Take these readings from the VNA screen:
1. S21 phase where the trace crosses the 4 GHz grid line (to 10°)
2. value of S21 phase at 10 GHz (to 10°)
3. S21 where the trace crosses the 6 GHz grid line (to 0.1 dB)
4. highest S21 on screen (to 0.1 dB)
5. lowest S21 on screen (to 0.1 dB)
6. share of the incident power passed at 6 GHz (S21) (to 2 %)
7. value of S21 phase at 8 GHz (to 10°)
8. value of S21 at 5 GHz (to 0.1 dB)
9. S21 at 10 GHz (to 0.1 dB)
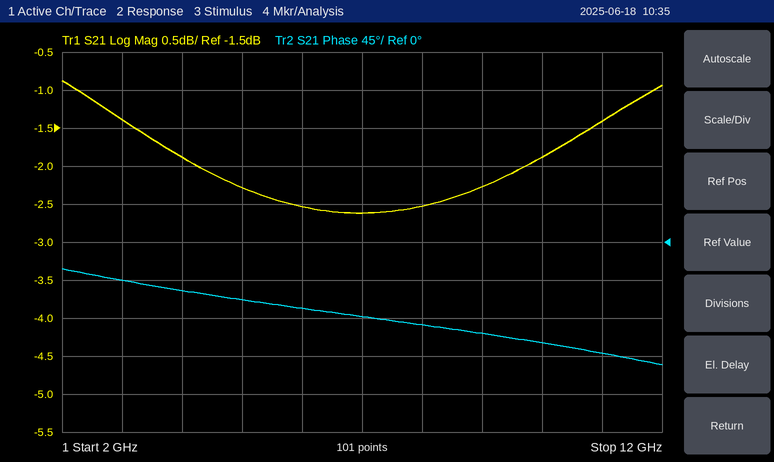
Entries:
-60°
-120°
-2.5 dB
-0.9 dB
-2.6 dB
56 %
-100°
-2.3 dB
-1.9 dB
